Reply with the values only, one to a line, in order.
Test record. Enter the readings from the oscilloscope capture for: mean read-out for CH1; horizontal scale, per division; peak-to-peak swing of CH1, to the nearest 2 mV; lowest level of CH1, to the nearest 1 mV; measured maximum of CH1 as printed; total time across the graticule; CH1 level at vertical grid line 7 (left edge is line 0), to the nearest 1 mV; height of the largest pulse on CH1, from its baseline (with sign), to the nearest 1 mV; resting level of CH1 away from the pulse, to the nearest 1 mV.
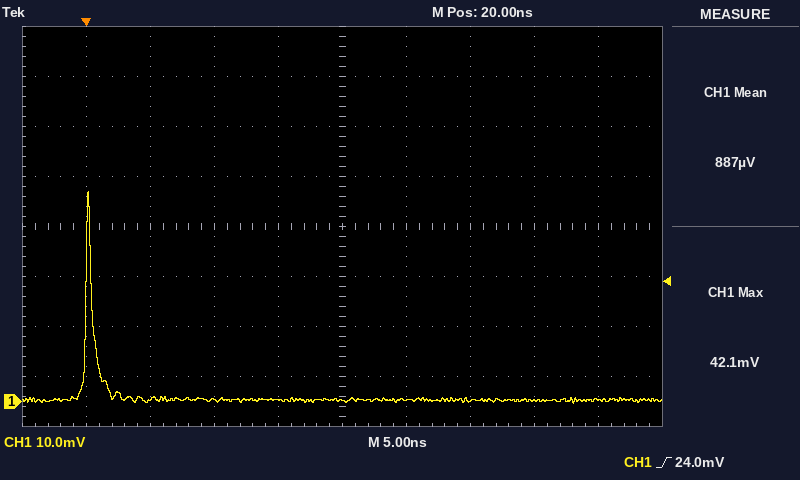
887 µV
5 ns
42 mV
0 mV
42.1 mV
50 ns
0 mV
+42 mV
0 mV
